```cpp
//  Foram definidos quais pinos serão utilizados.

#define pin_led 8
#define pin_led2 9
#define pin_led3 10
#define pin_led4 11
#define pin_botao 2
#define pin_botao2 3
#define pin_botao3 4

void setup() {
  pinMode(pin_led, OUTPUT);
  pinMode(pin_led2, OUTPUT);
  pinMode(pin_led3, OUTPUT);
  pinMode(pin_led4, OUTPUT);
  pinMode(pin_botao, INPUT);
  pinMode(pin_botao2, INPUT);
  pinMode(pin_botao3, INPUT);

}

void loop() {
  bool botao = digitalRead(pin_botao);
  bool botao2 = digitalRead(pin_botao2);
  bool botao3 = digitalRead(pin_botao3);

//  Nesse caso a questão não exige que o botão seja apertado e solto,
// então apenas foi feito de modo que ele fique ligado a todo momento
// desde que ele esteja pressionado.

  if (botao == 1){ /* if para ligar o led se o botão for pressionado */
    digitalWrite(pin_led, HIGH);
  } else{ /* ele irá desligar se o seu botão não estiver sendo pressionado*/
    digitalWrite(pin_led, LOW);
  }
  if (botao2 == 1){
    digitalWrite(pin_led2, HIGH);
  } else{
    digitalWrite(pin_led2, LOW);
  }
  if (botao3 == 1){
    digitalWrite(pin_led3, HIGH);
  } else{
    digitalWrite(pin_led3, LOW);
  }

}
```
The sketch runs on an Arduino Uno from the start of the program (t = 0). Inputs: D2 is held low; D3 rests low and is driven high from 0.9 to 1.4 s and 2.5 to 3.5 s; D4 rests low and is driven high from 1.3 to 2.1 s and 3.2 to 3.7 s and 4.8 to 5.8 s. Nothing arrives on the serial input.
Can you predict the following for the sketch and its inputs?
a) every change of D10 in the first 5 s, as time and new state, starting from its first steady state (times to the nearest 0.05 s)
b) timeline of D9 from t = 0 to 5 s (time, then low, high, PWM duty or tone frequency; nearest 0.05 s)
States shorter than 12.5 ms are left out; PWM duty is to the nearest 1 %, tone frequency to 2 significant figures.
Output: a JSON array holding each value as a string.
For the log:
["0 s low; 1.3 s high; 2.1 s low; 3.2 s high; 3.7 s low; 4.8 s high", "0 s low; 0.9 s high; 1.4 s low; 2.5 s high; 3.5 s low"]
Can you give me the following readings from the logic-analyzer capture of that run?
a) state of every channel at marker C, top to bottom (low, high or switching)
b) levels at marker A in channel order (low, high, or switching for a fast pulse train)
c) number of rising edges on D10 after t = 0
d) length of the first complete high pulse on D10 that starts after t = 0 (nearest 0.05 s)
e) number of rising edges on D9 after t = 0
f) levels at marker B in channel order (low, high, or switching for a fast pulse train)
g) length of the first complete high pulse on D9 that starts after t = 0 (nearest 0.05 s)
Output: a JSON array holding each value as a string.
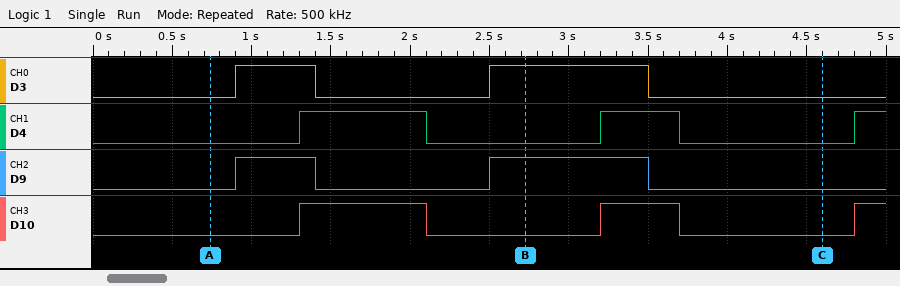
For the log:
["D3 low, D4 low, D9 low, D10 low", "D3 low, D4 low, D9 low, D10 low", "3", "0.80 s", "2", "D3 high, D4 low, D9 high, D10 low", "0.50 s"]
